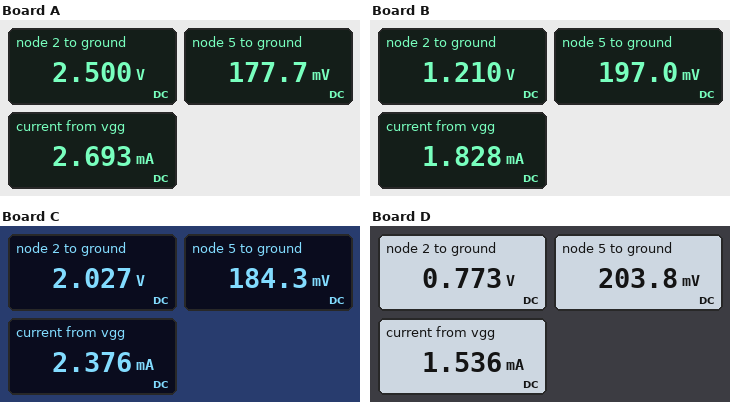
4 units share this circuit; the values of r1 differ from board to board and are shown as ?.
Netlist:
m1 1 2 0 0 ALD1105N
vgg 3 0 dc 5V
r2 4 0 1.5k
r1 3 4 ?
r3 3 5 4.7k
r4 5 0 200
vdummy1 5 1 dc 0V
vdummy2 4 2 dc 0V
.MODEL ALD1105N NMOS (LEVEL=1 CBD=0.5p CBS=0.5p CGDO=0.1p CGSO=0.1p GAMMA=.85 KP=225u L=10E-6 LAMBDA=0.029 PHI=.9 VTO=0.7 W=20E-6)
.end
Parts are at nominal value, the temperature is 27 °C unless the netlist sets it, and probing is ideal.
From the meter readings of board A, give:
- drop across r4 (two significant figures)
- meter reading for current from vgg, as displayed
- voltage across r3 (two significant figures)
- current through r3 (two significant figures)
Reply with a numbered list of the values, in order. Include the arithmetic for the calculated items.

1. 177.7 mV = 180 mV
2. 2.693 mA
3. 5 V - 177.7 mV = 4.8 V
4. (5 V - 177.7 mV) / 4.7 kΩ = 1.0 mA
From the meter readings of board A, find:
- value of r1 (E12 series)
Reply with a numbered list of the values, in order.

1. 1.5 kΩ
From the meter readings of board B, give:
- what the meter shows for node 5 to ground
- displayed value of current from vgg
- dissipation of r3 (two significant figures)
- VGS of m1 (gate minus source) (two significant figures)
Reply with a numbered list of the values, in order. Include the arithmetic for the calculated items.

1. 197.0 mV
2. 1.828 mA
3. (5 V - 197 mV)^2 / 4.7 kΩ = 4.9 mW
4. 1.21 V = 1.2 V
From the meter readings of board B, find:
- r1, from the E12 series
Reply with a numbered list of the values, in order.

1. 4.7 kΩ
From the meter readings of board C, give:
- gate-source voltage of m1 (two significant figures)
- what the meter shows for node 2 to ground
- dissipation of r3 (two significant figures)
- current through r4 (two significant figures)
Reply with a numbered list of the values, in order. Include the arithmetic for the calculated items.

1. 2.027 V = 2.0 V
2. 2.027 V
3. (5 V - 184.3 mV)^2 / 4.7 kΩ = 4.9 mW
4. (184.3 mV) / 200 Ω = 920 µA
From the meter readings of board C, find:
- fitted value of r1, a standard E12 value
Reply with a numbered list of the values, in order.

1. 2.2 kΩ
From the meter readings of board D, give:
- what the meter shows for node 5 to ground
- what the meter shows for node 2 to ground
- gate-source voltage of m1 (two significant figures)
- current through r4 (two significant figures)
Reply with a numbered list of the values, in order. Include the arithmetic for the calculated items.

1. 203.8 mV
2. 0.773 V
3. 773 mV = 770 mV
4. (203.8 mV) / 200 Ω = 1.0 mA
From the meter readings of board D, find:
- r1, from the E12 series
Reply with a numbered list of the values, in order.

1. 8.2 kΩ
